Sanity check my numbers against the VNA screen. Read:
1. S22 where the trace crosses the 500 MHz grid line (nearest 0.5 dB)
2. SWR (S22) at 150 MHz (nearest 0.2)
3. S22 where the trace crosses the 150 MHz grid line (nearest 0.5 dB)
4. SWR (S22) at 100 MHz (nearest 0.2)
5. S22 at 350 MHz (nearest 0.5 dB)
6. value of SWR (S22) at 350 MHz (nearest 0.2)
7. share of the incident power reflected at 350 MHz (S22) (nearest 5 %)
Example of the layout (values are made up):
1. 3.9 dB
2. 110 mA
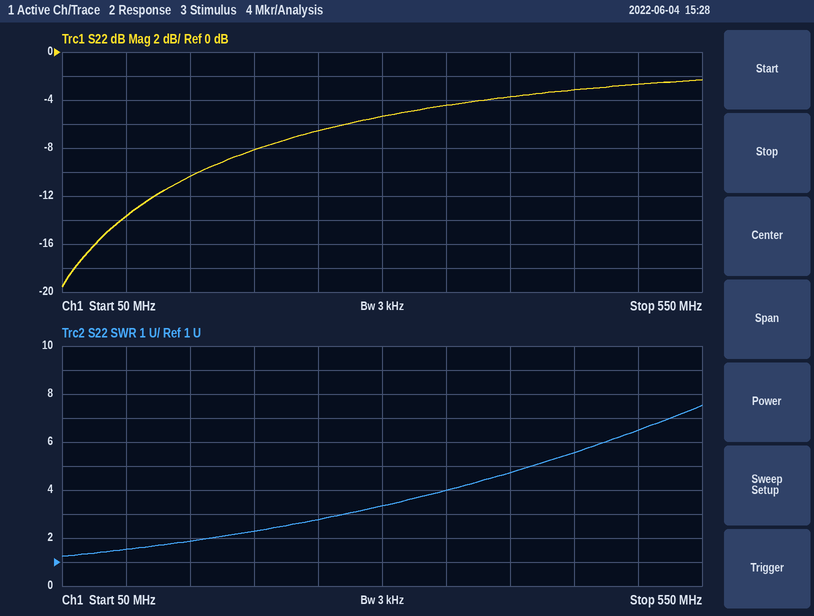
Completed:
1. -2.5 dB
2. 1.8
3. -10.5 dB
4. 1.6
5. -4.5 dB
6. 4.0
7. 35 %
